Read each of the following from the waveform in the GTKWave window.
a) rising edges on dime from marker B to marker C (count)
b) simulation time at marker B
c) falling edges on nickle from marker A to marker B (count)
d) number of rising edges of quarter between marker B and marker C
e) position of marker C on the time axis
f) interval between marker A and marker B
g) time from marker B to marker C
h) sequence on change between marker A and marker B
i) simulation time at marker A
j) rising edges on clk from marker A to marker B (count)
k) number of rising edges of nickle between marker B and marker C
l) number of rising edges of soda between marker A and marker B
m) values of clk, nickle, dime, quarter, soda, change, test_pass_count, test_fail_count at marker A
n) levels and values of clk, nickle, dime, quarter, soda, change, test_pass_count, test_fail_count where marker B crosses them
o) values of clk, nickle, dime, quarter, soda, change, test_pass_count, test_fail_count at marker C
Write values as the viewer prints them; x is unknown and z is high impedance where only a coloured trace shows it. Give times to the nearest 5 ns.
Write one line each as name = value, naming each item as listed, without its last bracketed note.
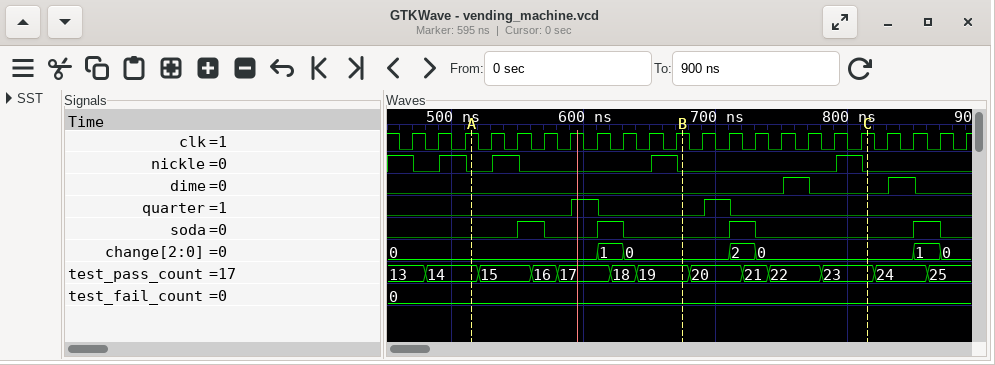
rising edges on dime from marker B to marker C = 1
simulation time at marker B = 675 ns
falling edges on nickle from marker A to marker B = 2
number of rising edges of quarter between marker B and marker C = 1
position of marker C on the time axis = 815 ns
interval between marker A and marker B = 160 ns
time from marker B to marker C = 140 ns
sequence on change between marker A and marker B = 0, 1, 0
simulation time at marker A = 515 ns
rising edges on clk from marker A to marker B = 8
number of rising edges of nickle between marker B and marker C = 1
number of rising edges of soda between marker A and marker B = 2
values of clk, nickle, dime, quarter, soda, change, test_pass_count, test_fail_count at marker A = clk=1, nickle=0, dime=0, quarter=0, soda=0, change=0, test_pass_count=14, test_fail_count=0
levels and values of clk, nickle, dime, quarter, soda, change, test_pass_count, test_fail_count where marker B crosses them = clk=1, nickle=0, dime=0, quarter=0, soda=0, change=0, test_pass_count=19, test_fail_count=0
values of clk, nickle, dime, quarter, soda, change, test_pass_count, test_fail_count at marker C = clk=1, nickle=0, dime=0, quarter=0, soda=0, change=0, test_pass_count=23, test_fail_count=0
